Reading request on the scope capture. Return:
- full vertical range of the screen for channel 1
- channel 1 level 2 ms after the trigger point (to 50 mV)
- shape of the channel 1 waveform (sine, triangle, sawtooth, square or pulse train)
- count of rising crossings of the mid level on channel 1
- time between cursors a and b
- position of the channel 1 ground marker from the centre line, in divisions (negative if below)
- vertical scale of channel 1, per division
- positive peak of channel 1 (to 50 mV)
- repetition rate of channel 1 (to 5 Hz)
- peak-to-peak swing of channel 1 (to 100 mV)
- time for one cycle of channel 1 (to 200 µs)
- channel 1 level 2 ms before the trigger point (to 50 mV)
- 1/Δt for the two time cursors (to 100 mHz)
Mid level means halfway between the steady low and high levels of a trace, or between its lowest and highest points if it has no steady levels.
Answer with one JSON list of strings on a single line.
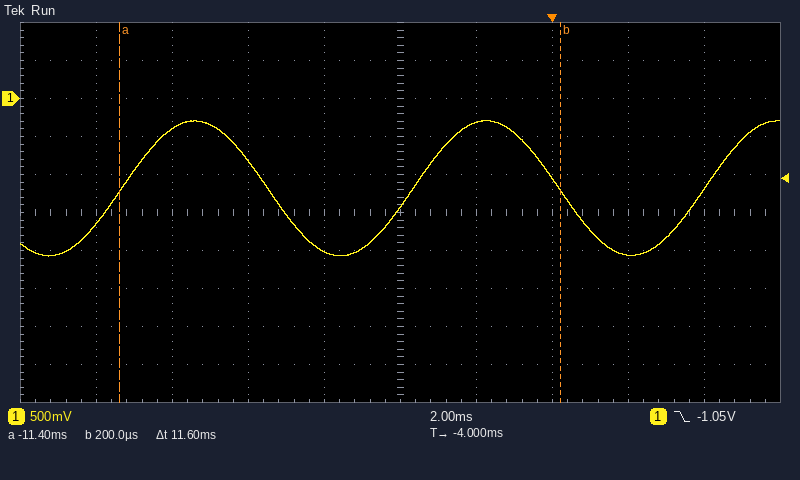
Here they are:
["5 V", "-2.05 V", "sine", "3", "11.6 ms", "+3.0 div", "500 mV", "-300 mV", "130 Hz", "1.80 V", "7.6 ms", "-300 mV", "86.2 Hz"]
